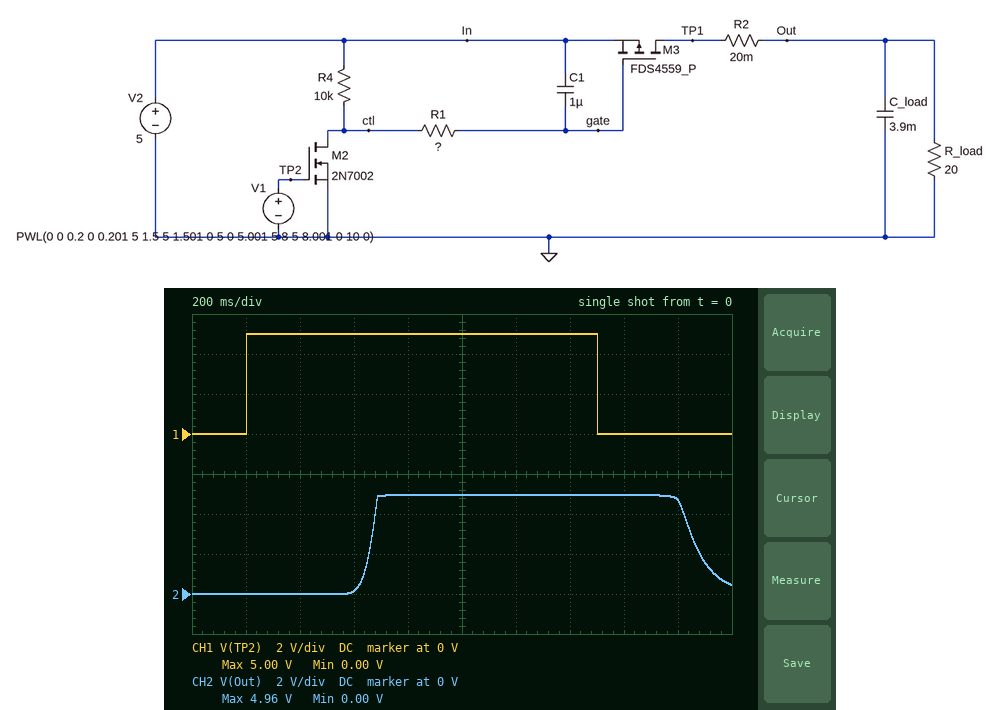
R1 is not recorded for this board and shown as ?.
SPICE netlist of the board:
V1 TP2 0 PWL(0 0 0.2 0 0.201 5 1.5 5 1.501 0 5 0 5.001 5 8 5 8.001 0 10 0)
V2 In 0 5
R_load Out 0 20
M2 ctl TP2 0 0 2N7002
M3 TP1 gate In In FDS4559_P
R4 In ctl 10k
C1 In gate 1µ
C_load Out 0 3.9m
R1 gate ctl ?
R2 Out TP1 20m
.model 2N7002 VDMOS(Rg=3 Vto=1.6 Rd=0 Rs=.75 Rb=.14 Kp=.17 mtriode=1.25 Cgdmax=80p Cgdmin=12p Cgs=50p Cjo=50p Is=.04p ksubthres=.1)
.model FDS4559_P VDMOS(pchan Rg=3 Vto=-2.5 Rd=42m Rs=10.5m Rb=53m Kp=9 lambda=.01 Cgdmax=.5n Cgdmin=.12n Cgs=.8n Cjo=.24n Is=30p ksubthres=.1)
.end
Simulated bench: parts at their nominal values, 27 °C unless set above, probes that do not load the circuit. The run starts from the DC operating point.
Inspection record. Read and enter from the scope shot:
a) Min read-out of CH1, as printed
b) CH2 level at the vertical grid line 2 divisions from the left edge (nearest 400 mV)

0.00 V
0 V
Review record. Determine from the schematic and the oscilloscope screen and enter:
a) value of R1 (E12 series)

560 kΩ
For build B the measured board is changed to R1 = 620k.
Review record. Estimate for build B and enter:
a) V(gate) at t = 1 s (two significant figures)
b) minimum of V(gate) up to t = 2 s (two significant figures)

1.4 V
620 mV
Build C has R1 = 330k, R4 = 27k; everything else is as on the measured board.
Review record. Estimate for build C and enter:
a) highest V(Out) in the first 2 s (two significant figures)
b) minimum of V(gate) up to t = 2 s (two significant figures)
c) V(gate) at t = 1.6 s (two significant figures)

5.0 V
98 mV
1.3 V
